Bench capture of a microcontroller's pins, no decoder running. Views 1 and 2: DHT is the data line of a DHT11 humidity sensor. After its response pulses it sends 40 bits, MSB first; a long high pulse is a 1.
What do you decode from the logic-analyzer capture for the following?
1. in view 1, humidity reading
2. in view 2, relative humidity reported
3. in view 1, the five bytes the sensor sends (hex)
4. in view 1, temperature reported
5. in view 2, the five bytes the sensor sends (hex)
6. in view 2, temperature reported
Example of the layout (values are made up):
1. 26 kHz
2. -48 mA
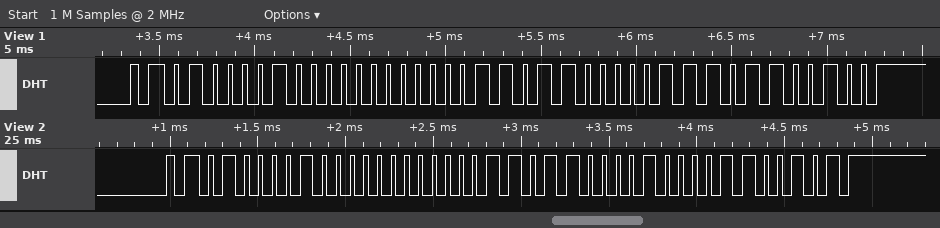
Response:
1. 66 %
2. 66 %
3. 42 00 1B 07 64
4. 27.7 °C
5. 42 00 1B 08 65
6. 27.8 °C
